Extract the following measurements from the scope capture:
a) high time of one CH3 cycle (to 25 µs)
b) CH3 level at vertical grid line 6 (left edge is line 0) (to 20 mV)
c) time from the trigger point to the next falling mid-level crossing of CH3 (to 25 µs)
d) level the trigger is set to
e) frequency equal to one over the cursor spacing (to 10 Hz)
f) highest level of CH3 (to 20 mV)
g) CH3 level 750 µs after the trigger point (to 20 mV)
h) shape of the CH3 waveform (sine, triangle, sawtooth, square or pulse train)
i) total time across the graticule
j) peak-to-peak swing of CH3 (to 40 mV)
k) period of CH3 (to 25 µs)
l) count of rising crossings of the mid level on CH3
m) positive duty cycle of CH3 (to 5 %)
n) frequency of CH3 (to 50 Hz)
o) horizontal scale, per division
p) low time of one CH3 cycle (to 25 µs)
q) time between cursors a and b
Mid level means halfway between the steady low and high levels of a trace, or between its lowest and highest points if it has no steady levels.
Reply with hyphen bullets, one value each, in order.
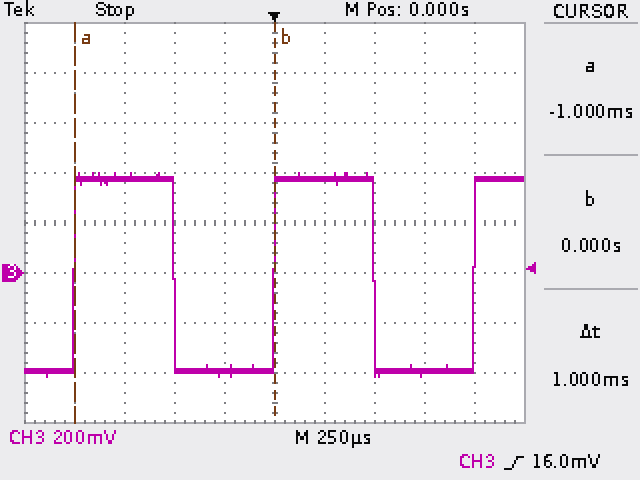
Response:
- 500 µs
- 380 mV
- 500 µs
- 16.0 mV
- 1.00 kHz
- 400 mV
- -400 mV
- square
- 2.5 ms
- 800 mV
- 1.000 ms
- 3
- 50 %
- 1.00 kHz
- 250 µs
- 500 µs
- 1 ms
